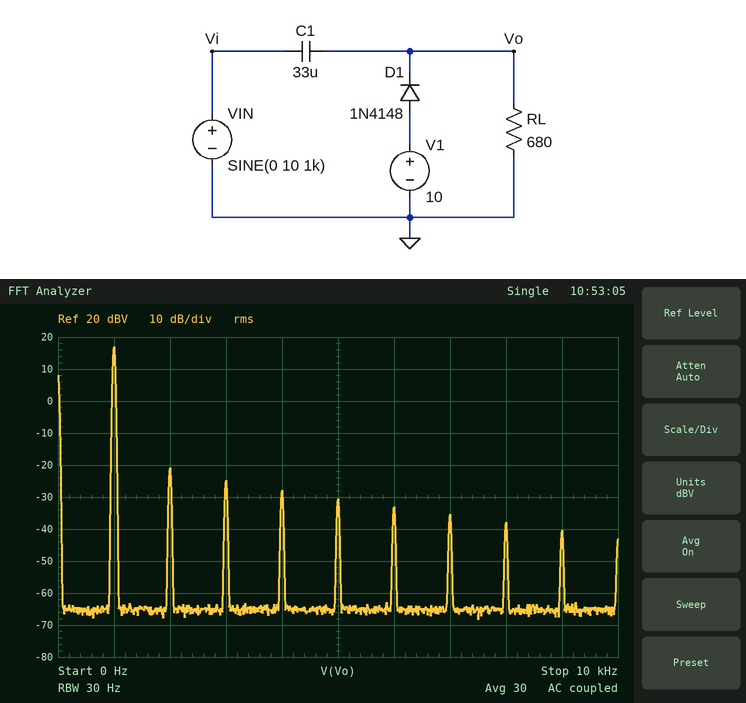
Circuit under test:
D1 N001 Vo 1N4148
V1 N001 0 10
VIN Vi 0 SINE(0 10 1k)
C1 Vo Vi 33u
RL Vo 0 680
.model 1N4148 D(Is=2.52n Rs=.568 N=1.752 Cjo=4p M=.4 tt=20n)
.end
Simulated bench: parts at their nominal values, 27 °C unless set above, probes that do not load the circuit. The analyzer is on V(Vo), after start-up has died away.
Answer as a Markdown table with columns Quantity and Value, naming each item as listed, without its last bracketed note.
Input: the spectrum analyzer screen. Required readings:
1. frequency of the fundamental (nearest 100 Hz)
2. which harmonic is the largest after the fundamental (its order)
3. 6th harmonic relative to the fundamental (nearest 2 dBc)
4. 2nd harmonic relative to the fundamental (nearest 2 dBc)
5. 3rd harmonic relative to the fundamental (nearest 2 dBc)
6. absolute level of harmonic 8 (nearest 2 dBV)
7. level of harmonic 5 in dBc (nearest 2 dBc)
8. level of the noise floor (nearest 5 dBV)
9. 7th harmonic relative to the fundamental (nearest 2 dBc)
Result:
| Quantity | Value |
|---|---|
| frequency of the fundamental | 1.0 kHz |
| which harmonic is the largest after the fundamental | 2 |
| 6th harmonic relative to the fundamental | -50 dBc |
| 2nd harmonic relative to the fundamental | -38 dBc |
| 3rd harmonic relative to the fundamental | -42 dBc |
| absolute level of harmonic 8 | -38 dBV |
| level of harmonic 5 in dBc | -48 dBc |
| level of the noise floor | -65 dBV |
| 7th harmonic relative to the fundamental | -52 dBc |
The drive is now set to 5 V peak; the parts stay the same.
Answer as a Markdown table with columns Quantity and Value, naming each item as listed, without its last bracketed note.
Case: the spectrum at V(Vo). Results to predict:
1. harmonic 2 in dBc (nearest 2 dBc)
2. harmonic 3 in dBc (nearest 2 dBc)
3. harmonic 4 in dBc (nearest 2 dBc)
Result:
| Quantity | Value |
|---|---|
| harmonic 2 in dBc | -34 dBc |
| harmonic 3 in dBc | -38 dBc |
| harmonic 4 in dBc | -42 dBc |
